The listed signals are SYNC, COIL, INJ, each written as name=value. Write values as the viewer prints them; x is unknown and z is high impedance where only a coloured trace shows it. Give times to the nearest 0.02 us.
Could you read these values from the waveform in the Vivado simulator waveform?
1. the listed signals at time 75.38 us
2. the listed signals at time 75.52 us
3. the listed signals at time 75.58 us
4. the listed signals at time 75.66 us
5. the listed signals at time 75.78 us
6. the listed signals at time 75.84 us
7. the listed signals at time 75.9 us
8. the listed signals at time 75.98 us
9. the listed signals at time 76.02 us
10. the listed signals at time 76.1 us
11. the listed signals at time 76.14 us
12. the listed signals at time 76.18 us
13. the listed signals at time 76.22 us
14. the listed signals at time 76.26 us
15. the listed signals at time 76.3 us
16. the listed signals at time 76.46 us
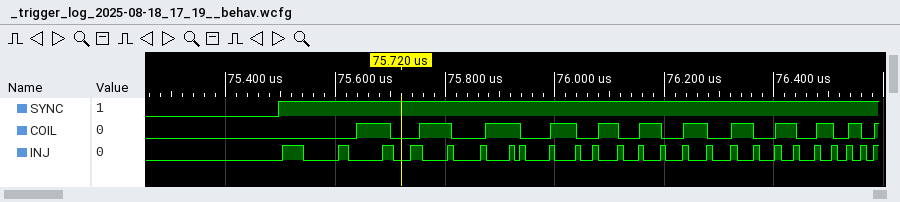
SYNC=0, COIL=0, INJ=0
SYNC=1, COIL=0, INJ=1
SYNC=1, COIL=0, INJ=0
SYNC=1, COIL=1, INJ=0
SYNC=1, COIL=1, INJ=0
SYNC=1, COIL=0, INJ=0
SYNC=1, COIL=1, INJ=0
SYNC=1, COIL=0, INJ=0
SYNC=1, COIL=1, INJ=0
SYNC=1, COIL=1, INJ=0
SYNC=1, COIL=0, INJ=0
SYNC=1, COIL=1, INJ=0
SYNC=1, COIL=0, INJ=0
SYNC=1, COIL=1, INJ=0
SYNC=1, COIL=0, INJ=0
SYNC=1, COIL=0, INJ=0
